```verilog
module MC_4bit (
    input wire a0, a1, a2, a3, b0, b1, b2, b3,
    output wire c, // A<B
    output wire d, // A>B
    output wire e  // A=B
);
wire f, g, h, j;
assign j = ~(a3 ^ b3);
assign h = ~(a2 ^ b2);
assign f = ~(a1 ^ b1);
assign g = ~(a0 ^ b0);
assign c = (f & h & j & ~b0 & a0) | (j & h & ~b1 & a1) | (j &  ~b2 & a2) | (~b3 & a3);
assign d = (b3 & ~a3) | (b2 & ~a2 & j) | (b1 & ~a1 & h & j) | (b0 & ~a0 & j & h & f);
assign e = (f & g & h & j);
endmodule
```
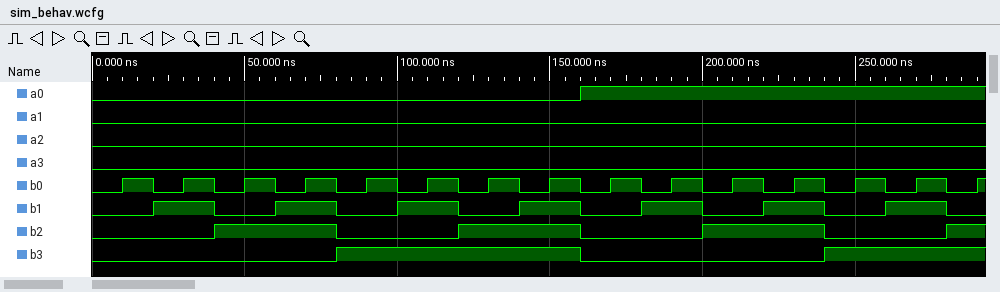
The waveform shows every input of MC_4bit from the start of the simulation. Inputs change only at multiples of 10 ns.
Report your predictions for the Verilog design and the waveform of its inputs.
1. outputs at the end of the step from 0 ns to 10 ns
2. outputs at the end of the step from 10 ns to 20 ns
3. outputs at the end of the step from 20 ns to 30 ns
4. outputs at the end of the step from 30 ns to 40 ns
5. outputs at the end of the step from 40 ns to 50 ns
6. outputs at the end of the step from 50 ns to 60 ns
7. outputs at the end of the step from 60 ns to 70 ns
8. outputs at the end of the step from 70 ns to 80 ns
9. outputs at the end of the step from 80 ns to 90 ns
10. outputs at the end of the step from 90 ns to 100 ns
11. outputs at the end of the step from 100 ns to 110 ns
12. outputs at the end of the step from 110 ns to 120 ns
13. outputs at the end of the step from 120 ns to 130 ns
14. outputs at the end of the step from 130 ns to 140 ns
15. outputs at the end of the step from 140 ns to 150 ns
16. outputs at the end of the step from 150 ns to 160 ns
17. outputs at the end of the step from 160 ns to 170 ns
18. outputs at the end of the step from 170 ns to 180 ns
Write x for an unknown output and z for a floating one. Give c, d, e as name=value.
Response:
c=0, d=0, e=1
c=0, d=1, e=0
c=0, d=1, e=0
c=0, d=1, e=0
c=0, d=1, e=0
c=0, d=1, e=0
c=0, d=1, e=0
c=0, d=1, e=0
c=0, d=1, e=0
c=0, d=1, e=0
c=0, d=1, e=0
c=0, d=1, e=0
c=0, d=1, e=0
c=0, d=1, e=0
c=0, d=1, e=0
c=0, d=1, e=0
c=1, d=0, e=0
c=0, d=0, e=1
